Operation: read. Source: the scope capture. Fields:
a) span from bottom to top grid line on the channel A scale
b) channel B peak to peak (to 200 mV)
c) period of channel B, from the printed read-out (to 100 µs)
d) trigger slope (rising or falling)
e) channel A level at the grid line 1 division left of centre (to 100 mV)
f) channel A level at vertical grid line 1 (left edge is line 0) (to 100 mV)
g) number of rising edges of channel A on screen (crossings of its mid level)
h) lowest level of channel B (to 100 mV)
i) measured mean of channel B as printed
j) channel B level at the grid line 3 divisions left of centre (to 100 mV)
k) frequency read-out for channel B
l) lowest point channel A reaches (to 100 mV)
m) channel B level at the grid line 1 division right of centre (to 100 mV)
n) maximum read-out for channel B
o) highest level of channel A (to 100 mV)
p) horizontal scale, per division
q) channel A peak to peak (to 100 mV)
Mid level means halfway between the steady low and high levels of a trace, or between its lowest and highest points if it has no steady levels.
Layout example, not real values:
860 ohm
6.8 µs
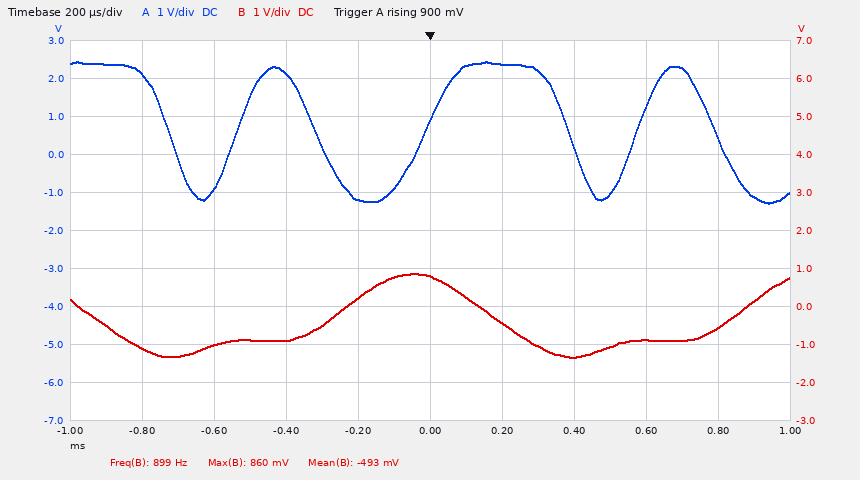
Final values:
10 V
2.2 V
1.1 ms
rising
-1.2 V
2.1 V
3
-1.3 V
-493 mV
-1.0 V
899 Hz
-1.3 V
-400 mV
860 mV
2.4 V
200 µs
3.7 V
